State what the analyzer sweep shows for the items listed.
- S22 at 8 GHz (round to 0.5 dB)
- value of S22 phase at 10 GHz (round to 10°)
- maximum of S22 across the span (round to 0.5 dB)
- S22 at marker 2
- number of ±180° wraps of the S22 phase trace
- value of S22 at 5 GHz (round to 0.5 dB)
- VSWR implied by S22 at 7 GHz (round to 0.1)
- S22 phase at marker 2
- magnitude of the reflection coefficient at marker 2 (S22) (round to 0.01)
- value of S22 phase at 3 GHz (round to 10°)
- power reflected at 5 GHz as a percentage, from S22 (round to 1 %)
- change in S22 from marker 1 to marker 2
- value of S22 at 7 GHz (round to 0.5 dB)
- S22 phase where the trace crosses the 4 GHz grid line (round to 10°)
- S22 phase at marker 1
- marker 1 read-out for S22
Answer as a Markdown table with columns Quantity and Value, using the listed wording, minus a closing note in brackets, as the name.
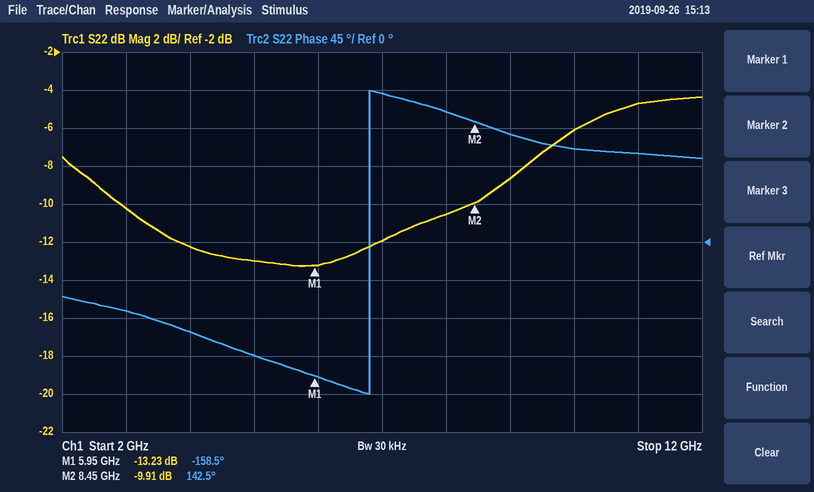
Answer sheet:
| Quantity | Value |
|---|---|
| S22 at 8 GHz | -10.5 dB |
| value of S22 phase at 10 GHz | 110° |
| maximum of S22 across the span | -4.5 dB |
| S22 at marker 2 | -9.91 dB |
| number of ±180° wraps of the S22 phase trace | 1 |
| value of S22 at 5 GHz | -13.0 dB |
| VSWR implied by S22 at 7 GHz | 1.7 |
| S22 phase at marker 2 | 142.5° |
| magnitude of the reflection coefficient at marker 2 (S22) | 0.32 |
| value of S22 phase at 3 GHz | -80° |
| power reflected at 5 GHz as a percentage, from S22 | 5 % |
| change in S22 from marker 1 to marker 2 | 3.32 dB |
| value of S22 at 7 GHz | -12.0 dB |
| S22 phase where the trace crosses the 4 GHz grid line | -110° |
| S22 phase at marker 1 | -158.5° |
| marker 1 read-out for S22 | -13.23 dB |
